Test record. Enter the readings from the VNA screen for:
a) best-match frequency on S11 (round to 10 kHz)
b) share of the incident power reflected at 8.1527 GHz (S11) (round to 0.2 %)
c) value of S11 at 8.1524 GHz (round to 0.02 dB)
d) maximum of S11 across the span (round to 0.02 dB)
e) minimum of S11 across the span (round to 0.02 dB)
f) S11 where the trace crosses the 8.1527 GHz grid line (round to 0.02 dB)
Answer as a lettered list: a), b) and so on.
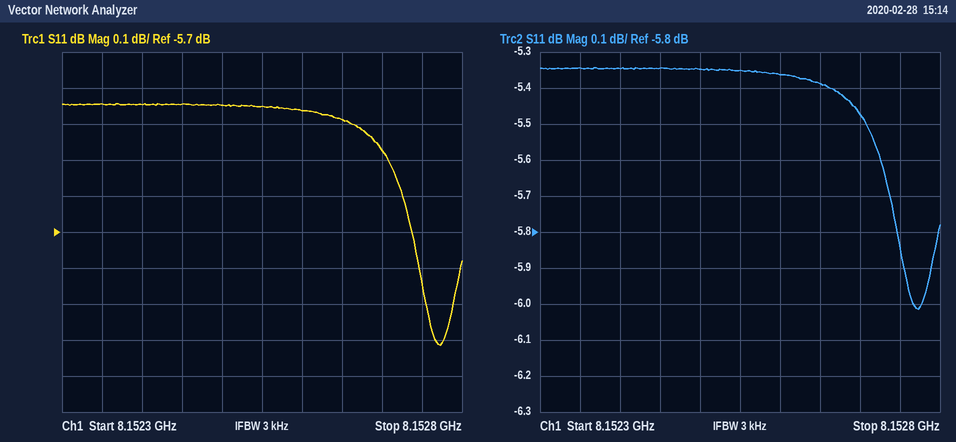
a) 8.15277 GHz
b) 28.4 %
c) -5.34 dB
d) -5.34 dB
e) -6.02 dB
f) -5.48 dB
